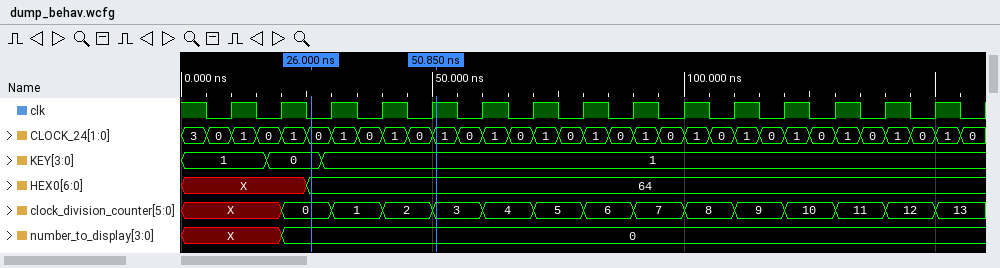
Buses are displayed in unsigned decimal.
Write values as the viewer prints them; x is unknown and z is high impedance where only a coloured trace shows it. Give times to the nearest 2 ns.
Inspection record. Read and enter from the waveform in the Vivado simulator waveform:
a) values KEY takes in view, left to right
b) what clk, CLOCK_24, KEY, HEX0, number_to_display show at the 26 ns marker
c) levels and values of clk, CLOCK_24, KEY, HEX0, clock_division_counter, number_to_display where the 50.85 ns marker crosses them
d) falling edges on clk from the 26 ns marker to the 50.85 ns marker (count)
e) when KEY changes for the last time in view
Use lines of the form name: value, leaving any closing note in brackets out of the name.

values KEY takes in view, left to right: 1, 0, 1
what clk, CLOCK_24, KEY, HEX0, number_to_display show at the 26 ns marker: clk=0, CLOCK_24=0, KEY=0, HEX0=64, number_to_display=0
levels and values of clk, CLOCK_24, KEY, HEX0, clock_division_counter, number_to_display where the 50.85 ns marker crosses them: clk=1, CLOCK_24=1, KEY=1, HEX0=64, clock_division_counter=3, number_to_display=0
falling edges on clk from the 26 ns marker to the 50.85 ns marker: 2
when KEY changes for the last time in view: 28 ns
